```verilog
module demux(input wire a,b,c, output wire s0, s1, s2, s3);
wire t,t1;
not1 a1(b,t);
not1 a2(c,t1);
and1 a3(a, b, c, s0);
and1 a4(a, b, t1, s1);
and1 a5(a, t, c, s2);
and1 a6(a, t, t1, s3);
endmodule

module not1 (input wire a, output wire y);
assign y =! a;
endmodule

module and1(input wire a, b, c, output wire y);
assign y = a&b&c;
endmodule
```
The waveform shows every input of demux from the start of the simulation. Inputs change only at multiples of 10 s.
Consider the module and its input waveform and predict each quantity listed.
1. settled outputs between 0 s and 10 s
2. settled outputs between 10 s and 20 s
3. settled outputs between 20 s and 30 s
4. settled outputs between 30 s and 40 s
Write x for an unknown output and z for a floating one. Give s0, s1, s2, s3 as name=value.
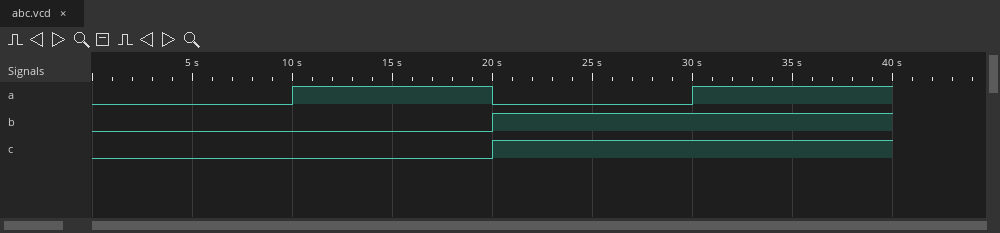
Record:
s0=0, s1=0, s2=0, s3=0
s0=0, s1=0, s2=0, s3=1
s0=0, s1=0, s2=0, s3=0
s0=1, s1=0, s2=0, s3=0
